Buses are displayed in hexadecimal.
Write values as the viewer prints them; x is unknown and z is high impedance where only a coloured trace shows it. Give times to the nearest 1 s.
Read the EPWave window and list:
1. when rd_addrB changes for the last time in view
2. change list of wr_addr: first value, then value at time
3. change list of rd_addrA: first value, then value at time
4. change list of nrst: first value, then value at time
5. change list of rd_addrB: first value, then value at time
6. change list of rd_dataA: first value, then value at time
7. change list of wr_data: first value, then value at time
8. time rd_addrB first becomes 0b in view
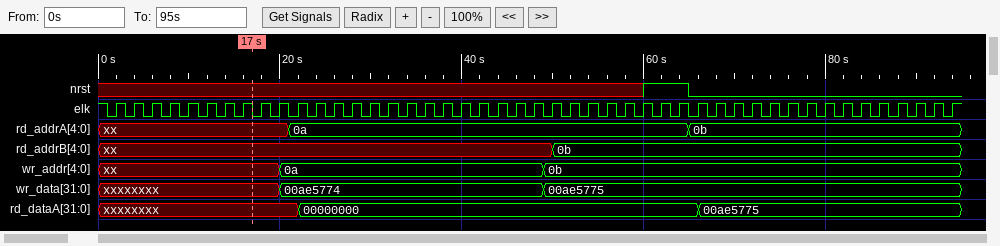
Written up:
50 s
xx, 0a at 20 s, 0b at 49 s
xx, 0a at 21 s, 0b at 65 s
x, 1 at 60 s, 0 at 65 s
xx, 0b at 50 s
xxxxxxxx, 00000000 at 22 s, 00ae5775 at 66 s
xxxxxxxx, 00ae5774 at 20 s, 00ae5775 at 49 s
50 s
